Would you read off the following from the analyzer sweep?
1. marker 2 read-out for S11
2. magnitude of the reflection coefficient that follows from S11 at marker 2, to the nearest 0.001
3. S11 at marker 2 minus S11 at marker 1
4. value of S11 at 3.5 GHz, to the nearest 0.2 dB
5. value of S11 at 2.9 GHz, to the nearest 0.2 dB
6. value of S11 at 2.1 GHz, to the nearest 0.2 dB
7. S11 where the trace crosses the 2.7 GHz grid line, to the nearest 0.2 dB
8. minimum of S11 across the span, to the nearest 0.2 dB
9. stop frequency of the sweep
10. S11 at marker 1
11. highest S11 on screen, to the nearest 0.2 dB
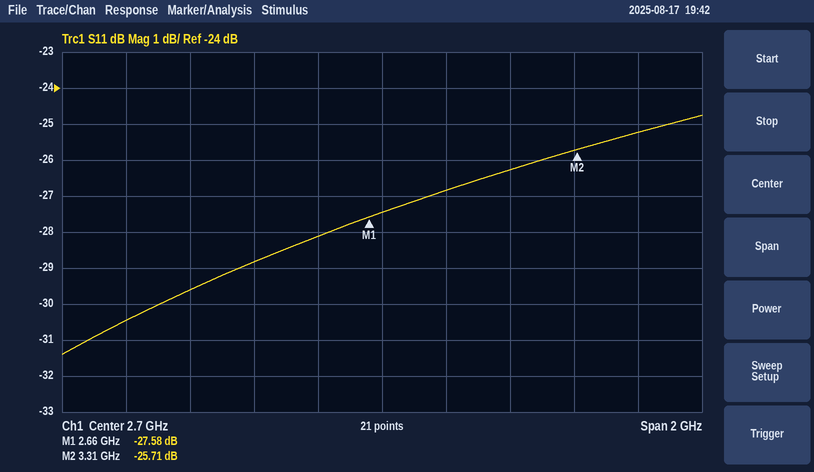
-25.71 dB
0.052
1.87 dB
-25.2 dB
-26.8 dB
-29.6 dB
-27.4 dB
-31.4 dB
3.7 GHz
-27.58 dB
-24.8 dB
